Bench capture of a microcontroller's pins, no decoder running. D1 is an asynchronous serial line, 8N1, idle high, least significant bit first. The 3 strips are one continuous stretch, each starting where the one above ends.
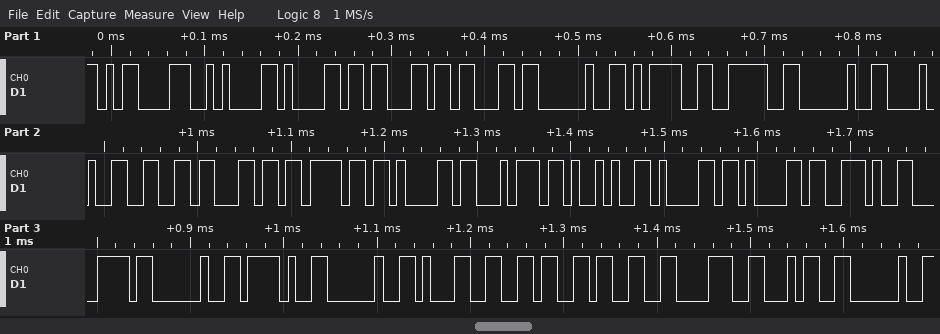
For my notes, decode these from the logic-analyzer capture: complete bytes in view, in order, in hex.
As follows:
0D 0A 61 63 63 20 3D 3E 20 28 66 6C 6F 61 74 29 61 61 2E 78 20 2F 20 31 36 33 38 34 20
